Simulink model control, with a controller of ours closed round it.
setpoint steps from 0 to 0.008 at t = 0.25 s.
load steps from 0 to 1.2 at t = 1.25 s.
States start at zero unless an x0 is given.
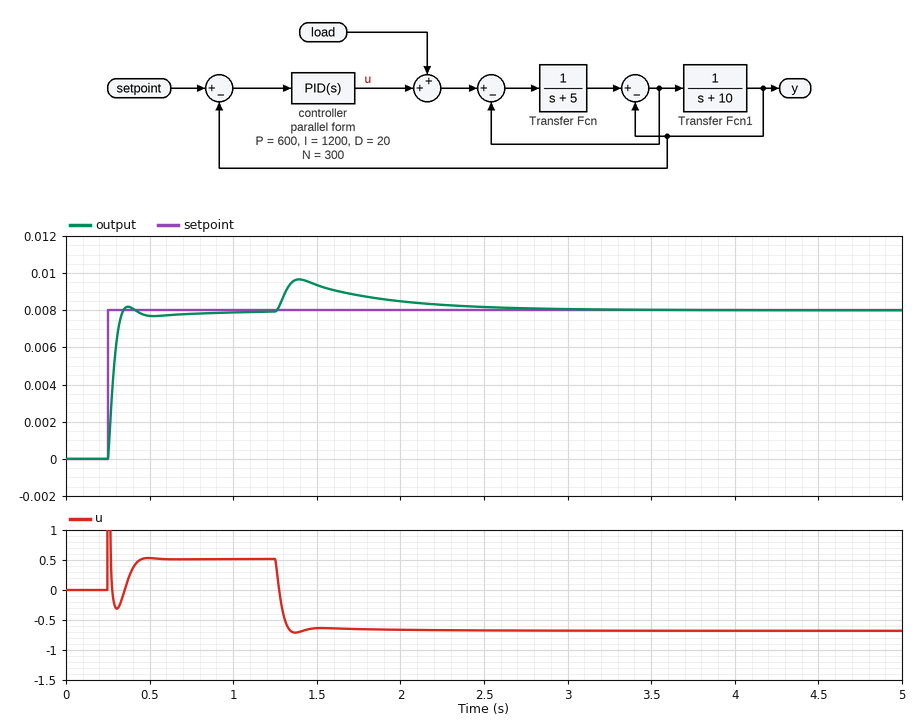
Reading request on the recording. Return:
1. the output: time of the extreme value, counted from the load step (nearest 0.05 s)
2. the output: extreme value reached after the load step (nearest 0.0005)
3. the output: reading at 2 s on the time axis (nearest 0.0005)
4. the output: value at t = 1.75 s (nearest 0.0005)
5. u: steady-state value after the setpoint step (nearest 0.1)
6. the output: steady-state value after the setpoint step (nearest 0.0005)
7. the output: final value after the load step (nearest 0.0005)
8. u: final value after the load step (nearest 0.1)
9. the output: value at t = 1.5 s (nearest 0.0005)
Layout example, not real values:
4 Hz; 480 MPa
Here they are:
0.15 s; 0.0095; 0.0085; 0.0090; 0.5; 0.0080; 0.0080; -0.7; 0.0095
